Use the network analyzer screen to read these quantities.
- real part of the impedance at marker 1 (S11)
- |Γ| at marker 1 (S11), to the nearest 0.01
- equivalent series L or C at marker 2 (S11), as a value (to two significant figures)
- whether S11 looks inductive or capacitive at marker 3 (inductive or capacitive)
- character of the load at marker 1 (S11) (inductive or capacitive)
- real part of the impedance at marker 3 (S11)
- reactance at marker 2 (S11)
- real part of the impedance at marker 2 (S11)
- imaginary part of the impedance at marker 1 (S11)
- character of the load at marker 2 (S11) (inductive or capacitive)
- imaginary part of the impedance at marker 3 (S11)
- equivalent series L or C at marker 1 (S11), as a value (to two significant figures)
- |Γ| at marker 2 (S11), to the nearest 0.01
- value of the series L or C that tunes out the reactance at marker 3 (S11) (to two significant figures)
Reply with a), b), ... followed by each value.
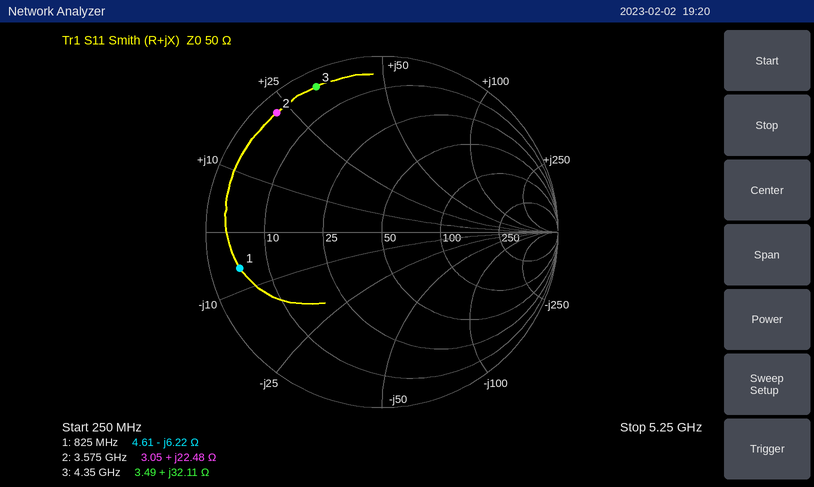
a) 4.61 Ω
b) 0.83
c) 1.0 nH
d) inductive
e) capacitive
f) 3.49 Ω
g) +22.48 Ω
h) 3.05 Ω
i) -6.22 Ω
j) inductive
k) +32.11 Ω
l) 31 pF
m) 0.90
n) 1.1 pF
